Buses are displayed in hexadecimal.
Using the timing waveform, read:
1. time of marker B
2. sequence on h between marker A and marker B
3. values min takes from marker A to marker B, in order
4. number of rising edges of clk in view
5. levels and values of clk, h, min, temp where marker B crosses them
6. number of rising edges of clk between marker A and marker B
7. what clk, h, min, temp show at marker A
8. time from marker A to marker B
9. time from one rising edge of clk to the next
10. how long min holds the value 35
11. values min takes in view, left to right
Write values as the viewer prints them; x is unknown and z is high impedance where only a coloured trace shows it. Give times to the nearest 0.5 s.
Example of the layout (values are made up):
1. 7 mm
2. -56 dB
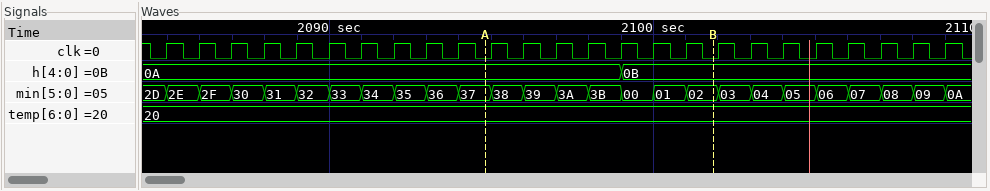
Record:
1. 2102 s
2. 0A, 0B
3. 37, 38, 39, 3A, 3B, 00, 01, 02
4. 25
5. clk=0, h=0B, min=02, temp=20
6. 7
7. clk=0, h=0A, min=37, temp=20
8. 7 s
9. 1 s
10. 1 s
11. 2D, 2E, 2F, 30, 31, 32, 33, 34, 35, 36, 37, 38, 39, 3A, 3B, 00, 01, 02, 03, 04, 05, 06, 07, 08, 09, 0A
